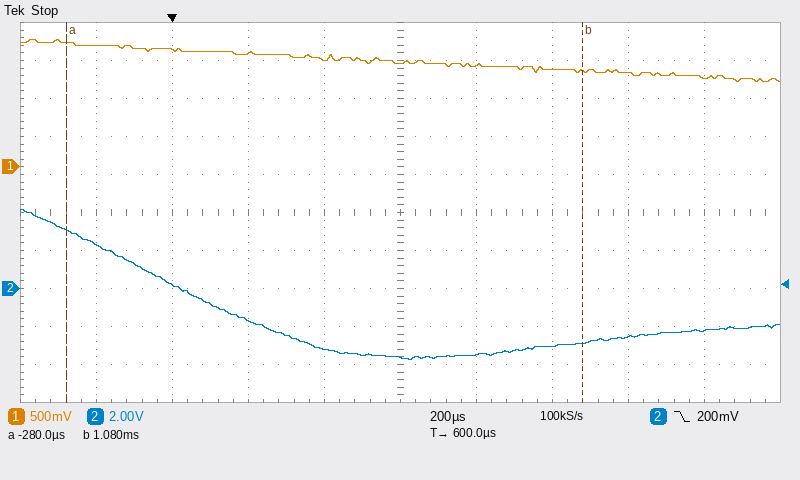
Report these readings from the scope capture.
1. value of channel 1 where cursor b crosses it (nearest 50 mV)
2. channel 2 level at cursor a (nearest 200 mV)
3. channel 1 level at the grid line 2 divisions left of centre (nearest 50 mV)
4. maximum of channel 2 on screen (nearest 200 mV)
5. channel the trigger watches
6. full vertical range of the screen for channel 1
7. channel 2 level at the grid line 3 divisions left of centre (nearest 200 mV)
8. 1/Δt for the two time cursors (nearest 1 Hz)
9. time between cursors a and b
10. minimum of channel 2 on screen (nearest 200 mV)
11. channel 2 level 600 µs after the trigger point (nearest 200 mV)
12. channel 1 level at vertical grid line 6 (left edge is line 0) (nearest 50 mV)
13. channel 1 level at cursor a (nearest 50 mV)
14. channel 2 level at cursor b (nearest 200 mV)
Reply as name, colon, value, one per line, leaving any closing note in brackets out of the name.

value of channel 1 where cursor b crosses it: 1.25 V
channel 2 level at cursor a: 3.0 V
channel 1 level at the grid line 2 divisions left of centre: 1.50 V
maximum of channel 2 on screen: 4.2 V
channel the trigger watches: channel 2
full vertical range of the screen for channel 1: 5 V
channel 2 level at the grid line 3 divisions left of centre: 200 mV
1/Δt for the two time cursors: 735 Hz
time between cursors a and b: 1.36 ms
minimum of channel 2 on screen: -3.8 V
channel 2 level 600 µs after the trigger point: -3.6 V
channel 1 level at vertical grid line 6 (left edge is line 0): 1.35 V
channel 1 level at cursor a: 1.65 V
channel 2 level at cursor b: -2.8 V
